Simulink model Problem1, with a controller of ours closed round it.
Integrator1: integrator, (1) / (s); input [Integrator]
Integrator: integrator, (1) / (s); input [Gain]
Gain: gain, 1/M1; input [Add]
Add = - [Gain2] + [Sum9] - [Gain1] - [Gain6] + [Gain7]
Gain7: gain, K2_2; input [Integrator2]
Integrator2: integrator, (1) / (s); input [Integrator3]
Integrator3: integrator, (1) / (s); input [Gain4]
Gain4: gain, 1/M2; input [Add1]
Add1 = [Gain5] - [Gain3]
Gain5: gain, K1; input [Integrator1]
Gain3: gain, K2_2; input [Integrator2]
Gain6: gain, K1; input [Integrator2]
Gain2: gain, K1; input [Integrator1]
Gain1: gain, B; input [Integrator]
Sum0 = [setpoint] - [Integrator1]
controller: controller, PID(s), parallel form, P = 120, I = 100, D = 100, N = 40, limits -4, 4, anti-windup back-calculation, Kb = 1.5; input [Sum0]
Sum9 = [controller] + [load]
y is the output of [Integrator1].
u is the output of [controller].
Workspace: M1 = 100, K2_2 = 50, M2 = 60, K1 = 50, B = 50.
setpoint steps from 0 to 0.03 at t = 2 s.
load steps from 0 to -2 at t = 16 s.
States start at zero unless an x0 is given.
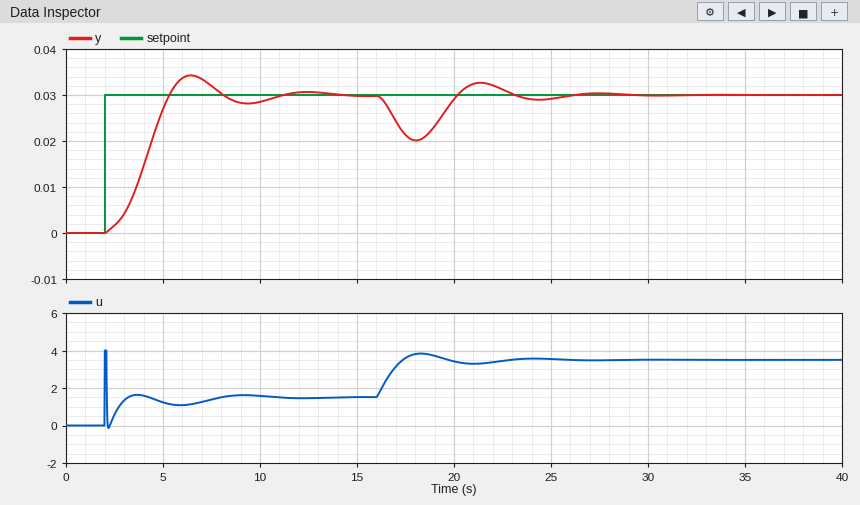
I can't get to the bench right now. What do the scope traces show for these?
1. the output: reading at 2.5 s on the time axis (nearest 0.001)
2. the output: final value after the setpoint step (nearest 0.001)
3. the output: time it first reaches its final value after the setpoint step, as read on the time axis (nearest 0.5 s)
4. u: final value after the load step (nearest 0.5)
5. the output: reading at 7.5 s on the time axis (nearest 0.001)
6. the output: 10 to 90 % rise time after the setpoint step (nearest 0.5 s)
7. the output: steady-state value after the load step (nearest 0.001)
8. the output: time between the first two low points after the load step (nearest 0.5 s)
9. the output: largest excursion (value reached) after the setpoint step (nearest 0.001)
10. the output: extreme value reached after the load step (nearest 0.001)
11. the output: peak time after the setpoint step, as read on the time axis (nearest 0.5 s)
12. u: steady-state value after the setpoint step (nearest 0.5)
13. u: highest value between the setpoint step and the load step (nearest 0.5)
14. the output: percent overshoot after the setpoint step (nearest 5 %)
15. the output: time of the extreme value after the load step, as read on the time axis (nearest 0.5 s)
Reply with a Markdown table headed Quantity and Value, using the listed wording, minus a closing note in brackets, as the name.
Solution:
| Quantity | Value |
|---|---|
| the output: reading at 2.5 s on the time axis | 0.002 |
| the output: final value after the setpoint step | 0.030 |
| the output: time it first reaches its final value after the setpoint step, as read on the time axis | 5.5 s |
| u: final value after the load step | 3.5 |
| the output: reading at 7.5 s on the time axis | 0.032 |
| the output: 10 to 90 % rise time after the setpoint step | 2.0 s |
| the output: steady-state value after the load step | 0.030 |
| the output: time between the first two low points after the load step | 6.5 s |
| the output: largest excursion (value reached) after the setpoint step | 0.034 |
| the output: extreme value reached after the load step | 0.020 |
| the output: peak time after the setpoint step, as read on the time axis | 6.5 s |
| u: steady-state value after the setpoint step | 1.5 |
| u: highest value between the setpoint step and the load step | 4.0 |
| the output: percent overshoot after the setpoint step | 15 % |
| the output: time of the extreme value after the load step, as read on the time axis | 18.0 s |
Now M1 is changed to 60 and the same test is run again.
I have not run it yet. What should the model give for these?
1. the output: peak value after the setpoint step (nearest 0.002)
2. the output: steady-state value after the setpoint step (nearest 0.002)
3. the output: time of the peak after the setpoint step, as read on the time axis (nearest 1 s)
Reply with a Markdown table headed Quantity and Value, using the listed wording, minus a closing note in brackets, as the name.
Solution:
| Quantity | Value |
|---|---|
| the output: peak value after the setpoint step | 0.032 |
| the output: steady-state value after the setpoint step | 0.030 |
| the output: time of the peak after the setpoint step, as read on the time axis | 7 s |
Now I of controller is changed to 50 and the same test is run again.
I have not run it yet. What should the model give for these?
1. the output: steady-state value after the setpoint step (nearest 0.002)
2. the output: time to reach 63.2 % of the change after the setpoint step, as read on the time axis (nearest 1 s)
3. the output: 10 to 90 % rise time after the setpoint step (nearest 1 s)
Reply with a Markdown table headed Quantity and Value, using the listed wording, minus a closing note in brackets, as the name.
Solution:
| Quantity | Value |
|---|---|
| the output: steady-state value after the setpoint step | 0.030 |
| the output: time to reach 63.2 % of the change after the setpoint step, as read on the time axis | 6 s |
| the output: 10 to 90 % rise time after the setpoint step | 5 s |
